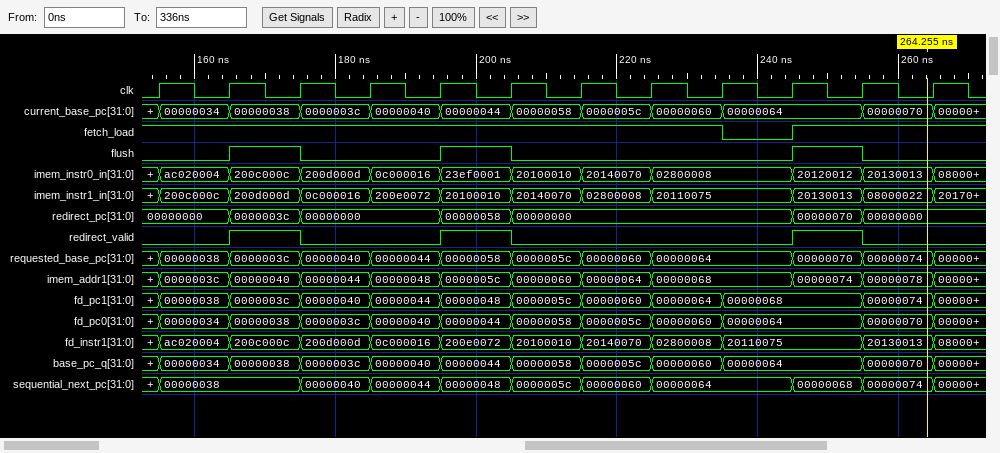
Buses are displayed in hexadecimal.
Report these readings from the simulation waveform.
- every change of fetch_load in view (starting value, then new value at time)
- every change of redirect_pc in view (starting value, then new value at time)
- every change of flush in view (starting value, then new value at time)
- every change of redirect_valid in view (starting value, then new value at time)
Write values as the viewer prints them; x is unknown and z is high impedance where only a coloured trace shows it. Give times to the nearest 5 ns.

1, 0 at 235 ns, 1 at 245 ns
00000000, 0000003c at 165 ns, 00000000 at 175 ns, 00000058 at 195 ns, 00000000 at 205 ns, 00000070 at 245 ns, 00000000 at 255 ns
0, 1 at 165 ns, 0 at 175 ns, 1 at 195 ns, 0 at 205 ns, 1 at 245 ns, 0 at 255 ns
0, 1 at 165 ns, 0 at 175 ns, 1 at 195 ns, 0 at 205 ns, 1 at 245 ns, 0 at 255 ns
